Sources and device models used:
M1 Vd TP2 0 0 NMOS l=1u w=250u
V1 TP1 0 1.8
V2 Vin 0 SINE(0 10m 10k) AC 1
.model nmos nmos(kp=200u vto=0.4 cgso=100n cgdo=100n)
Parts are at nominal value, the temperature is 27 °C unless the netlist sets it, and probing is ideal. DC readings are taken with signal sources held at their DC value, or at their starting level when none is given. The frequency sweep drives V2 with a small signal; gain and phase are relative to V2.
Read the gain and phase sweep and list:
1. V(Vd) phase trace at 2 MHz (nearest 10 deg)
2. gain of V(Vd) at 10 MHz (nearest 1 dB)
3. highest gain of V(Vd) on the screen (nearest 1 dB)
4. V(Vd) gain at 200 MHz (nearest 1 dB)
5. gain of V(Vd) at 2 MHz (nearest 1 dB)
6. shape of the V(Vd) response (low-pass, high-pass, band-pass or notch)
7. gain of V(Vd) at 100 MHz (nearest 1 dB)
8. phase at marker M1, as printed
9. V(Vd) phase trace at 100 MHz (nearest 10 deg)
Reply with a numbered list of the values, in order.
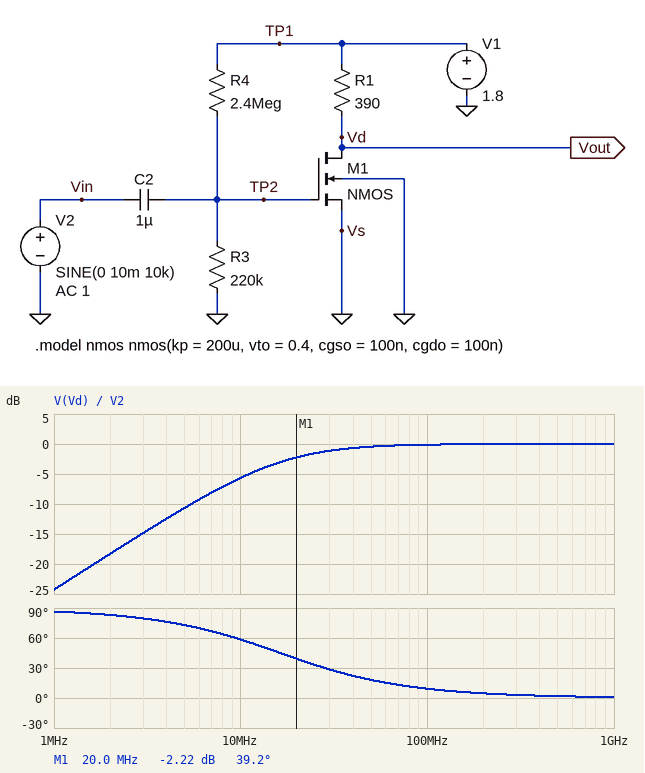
1. 80 deg
2. -6 dB
3. 0 dB
4. 0 dB
5. -18 dB
6. high-pass
7. 0 dB
8. 39.2 deg
9. 10 deg
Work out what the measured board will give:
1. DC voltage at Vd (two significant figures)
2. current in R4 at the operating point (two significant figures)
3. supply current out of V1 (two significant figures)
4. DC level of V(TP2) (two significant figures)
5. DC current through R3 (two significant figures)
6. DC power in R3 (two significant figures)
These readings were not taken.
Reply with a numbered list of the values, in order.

1. 1.8 V
2. 690 nA
3. 690 nA
4. 150 mV
5. 690 nA
6. 100 nW
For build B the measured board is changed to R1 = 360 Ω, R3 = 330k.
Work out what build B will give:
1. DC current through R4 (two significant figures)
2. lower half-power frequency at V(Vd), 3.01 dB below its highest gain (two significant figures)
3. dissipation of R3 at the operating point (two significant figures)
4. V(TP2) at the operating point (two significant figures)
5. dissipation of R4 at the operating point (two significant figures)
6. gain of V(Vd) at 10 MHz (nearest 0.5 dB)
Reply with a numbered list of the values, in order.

1. 660 nA
2. 18 MHz
3. 140 nW
4. 220 mV
5. 1.0 µW
6. -6.0 dB
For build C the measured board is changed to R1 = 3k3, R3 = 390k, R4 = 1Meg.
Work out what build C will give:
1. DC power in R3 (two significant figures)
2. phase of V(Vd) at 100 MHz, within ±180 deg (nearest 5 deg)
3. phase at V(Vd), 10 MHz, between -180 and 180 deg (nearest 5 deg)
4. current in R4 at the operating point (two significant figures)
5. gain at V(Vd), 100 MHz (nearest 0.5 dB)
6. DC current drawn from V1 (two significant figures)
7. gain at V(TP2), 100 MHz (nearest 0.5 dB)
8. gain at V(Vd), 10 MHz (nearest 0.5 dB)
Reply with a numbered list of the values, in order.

1. 650 nW
2. 20 deg
3. 85 deg
4. 1.3 µA
5. 0.5 dB
6. 280 µA
7. 0 dB
8. 10.5 dB
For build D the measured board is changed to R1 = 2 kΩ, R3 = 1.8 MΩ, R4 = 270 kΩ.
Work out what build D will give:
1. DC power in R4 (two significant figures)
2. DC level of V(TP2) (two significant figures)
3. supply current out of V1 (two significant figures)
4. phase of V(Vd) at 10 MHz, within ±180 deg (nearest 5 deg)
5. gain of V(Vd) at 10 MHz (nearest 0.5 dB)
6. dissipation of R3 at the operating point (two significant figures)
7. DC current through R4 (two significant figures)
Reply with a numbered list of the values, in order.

1. 200 nW
2. 1.6 V
3. 890 µA
4. 115 deg
5. -30.5 dB
6. 1.4 µW
7. 870 nA
